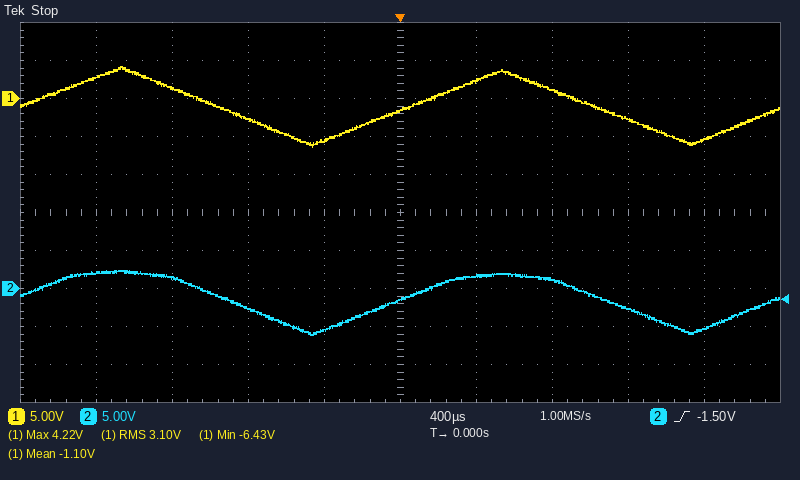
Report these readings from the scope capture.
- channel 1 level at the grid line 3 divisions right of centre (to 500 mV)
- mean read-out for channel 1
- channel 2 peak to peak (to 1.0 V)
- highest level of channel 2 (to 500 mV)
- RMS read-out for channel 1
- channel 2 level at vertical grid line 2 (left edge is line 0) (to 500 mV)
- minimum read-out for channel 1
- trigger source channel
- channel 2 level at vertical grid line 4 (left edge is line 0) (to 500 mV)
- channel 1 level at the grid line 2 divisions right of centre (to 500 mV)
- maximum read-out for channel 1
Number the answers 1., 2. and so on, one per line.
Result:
1. -3.0 V
2. -1.10 V
3. 9.0 V
4. 2.5 V
5. 3.10 V
6. 1.5 V
7. -6.43 V
8. channel 2
9. -5.5 V
10. 1.0 V
11. 4.22 V
